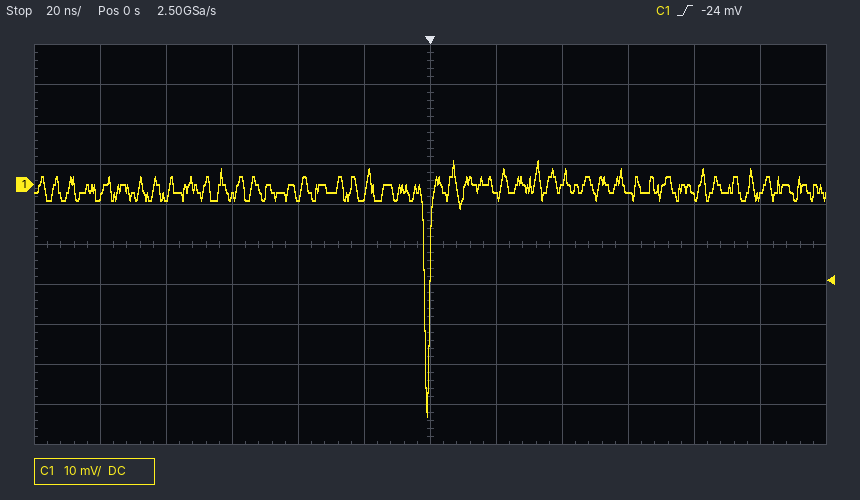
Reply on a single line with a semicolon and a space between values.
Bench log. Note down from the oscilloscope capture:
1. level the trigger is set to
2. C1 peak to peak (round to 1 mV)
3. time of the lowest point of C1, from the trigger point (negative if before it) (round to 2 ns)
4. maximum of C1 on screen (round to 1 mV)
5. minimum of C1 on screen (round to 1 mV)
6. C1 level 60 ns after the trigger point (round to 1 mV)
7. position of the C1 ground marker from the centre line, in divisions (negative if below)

-24 mV; 64 mV; 0 ns; 6 mV; -58 mV; -2 mV; +1.5 div
